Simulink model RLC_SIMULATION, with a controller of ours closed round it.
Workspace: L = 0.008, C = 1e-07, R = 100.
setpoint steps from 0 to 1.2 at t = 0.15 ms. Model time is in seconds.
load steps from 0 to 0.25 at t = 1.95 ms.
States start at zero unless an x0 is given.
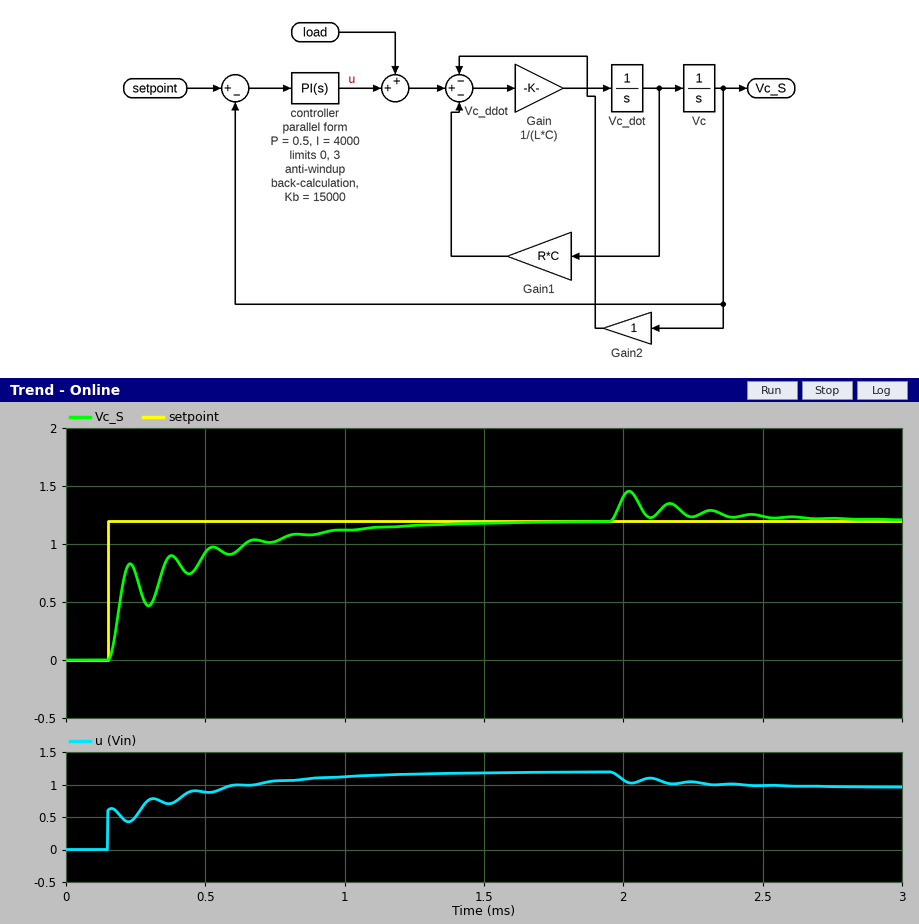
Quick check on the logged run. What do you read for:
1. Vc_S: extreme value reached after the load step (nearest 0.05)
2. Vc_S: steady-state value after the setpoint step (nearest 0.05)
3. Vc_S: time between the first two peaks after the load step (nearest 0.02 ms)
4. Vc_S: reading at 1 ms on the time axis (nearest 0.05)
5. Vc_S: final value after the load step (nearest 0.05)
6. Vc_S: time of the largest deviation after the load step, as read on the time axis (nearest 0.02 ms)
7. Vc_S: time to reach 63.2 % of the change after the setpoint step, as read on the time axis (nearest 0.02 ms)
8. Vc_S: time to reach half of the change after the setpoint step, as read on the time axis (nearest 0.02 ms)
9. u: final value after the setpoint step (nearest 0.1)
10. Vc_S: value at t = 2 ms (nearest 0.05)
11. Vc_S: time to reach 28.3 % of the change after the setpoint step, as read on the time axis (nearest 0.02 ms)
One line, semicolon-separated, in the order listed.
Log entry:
1.45; 1.20; 0.14 ms; 1.10; 1.20; 2.02 ms; 0.22 ms; 0.20 ms; 1.2; 1.40; 0.18 ms
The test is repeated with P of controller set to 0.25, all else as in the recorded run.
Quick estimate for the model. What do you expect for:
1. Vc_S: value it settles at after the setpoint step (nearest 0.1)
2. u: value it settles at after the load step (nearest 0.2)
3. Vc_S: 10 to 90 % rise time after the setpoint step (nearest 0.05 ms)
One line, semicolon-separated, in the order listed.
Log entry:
1.2; 1.0; 0.65 ms
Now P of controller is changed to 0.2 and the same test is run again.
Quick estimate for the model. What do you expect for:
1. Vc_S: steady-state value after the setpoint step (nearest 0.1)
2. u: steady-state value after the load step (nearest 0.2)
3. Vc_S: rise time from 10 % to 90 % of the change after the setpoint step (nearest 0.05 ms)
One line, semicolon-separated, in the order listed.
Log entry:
1.2; 1.0; 0.55 ms
